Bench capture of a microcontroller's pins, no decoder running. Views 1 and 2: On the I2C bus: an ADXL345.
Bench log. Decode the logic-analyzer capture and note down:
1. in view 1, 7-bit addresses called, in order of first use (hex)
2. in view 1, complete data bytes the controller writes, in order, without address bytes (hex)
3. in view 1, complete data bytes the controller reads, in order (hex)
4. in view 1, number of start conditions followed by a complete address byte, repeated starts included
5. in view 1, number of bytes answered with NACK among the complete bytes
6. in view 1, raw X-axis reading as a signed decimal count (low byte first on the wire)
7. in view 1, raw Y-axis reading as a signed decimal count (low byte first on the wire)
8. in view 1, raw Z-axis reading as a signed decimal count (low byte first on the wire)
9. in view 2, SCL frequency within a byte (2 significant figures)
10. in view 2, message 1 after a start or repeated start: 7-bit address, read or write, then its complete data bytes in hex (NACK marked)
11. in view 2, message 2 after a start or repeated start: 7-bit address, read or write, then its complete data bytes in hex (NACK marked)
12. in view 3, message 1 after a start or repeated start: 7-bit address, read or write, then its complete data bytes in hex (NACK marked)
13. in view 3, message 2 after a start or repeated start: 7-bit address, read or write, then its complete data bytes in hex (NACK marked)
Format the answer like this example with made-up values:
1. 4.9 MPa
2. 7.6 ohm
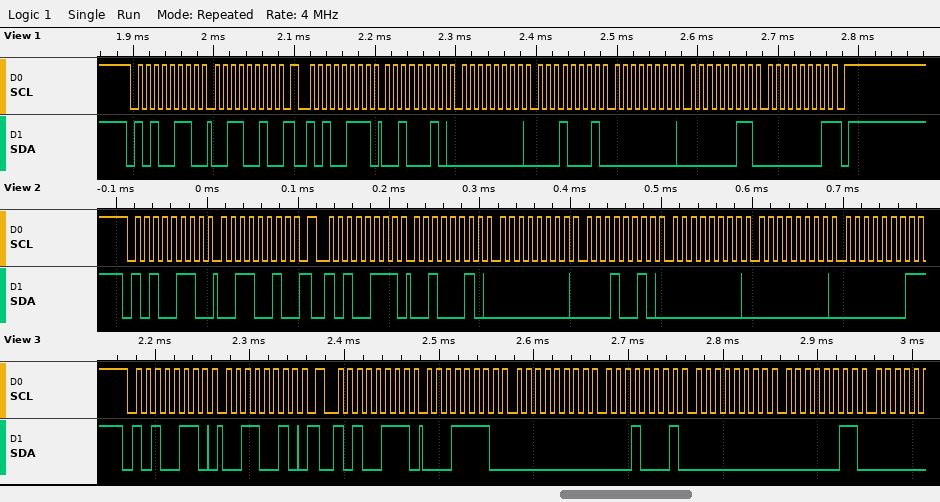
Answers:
1. 0x53
2. 32
3. 22 00 11 00 03 01
4. 2
5. 1
6. 34
7. 17
8. 259
9. 100 kHz
10. 0x53 write: 32
11. 0x53 read: 22 00 12 00 00 01 NACK
12. 0x53 write: 32
13. 0x53 read: 1E 00 11 00 03
